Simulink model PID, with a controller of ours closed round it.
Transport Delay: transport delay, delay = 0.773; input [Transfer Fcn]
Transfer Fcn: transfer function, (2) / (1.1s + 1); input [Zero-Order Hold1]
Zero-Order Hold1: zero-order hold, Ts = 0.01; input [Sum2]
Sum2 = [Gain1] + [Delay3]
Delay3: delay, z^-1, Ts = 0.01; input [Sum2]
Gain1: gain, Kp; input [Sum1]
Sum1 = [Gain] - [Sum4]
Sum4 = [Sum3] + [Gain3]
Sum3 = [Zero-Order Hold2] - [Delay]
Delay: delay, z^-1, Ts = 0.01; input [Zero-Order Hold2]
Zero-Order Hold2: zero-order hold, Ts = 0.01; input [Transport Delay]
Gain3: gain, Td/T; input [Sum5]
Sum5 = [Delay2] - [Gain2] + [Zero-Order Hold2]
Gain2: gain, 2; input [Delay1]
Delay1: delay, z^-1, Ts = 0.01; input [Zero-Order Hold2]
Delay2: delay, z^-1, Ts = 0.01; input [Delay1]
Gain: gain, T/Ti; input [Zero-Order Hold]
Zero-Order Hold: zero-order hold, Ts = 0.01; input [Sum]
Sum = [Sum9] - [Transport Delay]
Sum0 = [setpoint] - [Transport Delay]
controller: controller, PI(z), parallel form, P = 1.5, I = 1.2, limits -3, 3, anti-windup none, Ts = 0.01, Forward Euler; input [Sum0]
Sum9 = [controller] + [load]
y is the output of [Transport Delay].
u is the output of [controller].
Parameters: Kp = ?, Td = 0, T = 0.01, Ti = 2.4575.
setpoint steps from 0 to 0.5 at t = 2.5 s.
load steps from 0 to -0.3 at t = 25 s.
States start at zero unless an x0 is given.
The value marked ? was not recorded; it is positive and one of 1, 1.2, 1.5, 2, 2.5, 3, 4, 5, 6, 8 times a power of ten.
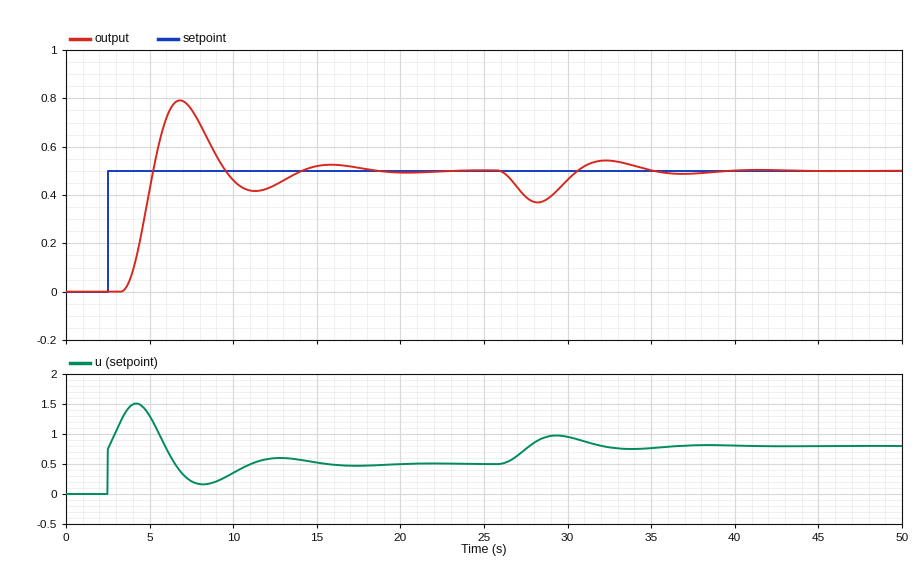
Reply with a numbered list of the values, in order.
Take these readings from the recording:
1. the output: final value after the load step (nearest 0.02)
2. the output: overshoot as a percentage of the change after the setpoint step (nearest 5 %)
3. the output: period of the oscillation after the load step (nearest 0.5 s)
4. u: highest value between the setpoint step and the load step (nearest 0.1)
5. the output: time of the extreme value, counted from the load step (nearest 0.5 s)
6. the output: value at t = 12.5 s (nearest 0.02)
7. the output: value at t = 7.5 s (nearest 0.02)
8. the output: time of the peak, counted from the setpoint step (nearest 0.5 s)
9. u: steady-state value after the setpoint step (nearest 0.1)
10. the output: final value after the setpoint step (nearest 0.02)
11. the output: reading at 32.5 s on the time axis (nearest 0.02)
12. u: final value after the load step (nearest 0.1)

1. 0.50
2. 60 %
3. 8.5 s
4. 1.5
5. 3.0 s
6. 0.44
7. 0.76
8. 4.5 s
9. 0.5
10. 0.50
11. 0.54
12. 0.8
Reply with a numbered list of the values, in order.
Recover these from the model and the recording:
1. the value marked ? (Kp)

1. 0.6
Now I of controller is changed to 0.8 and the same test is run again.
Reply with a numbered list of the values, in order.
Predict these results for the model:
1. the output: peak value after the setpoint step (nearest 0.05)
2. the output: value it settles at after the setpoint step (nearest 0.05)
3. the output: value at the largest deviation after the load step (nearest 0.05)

1. 0.65
2. 0.50
3. 0.35
